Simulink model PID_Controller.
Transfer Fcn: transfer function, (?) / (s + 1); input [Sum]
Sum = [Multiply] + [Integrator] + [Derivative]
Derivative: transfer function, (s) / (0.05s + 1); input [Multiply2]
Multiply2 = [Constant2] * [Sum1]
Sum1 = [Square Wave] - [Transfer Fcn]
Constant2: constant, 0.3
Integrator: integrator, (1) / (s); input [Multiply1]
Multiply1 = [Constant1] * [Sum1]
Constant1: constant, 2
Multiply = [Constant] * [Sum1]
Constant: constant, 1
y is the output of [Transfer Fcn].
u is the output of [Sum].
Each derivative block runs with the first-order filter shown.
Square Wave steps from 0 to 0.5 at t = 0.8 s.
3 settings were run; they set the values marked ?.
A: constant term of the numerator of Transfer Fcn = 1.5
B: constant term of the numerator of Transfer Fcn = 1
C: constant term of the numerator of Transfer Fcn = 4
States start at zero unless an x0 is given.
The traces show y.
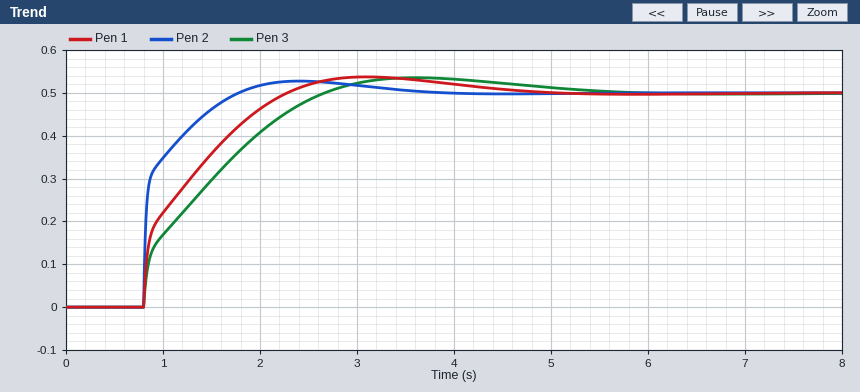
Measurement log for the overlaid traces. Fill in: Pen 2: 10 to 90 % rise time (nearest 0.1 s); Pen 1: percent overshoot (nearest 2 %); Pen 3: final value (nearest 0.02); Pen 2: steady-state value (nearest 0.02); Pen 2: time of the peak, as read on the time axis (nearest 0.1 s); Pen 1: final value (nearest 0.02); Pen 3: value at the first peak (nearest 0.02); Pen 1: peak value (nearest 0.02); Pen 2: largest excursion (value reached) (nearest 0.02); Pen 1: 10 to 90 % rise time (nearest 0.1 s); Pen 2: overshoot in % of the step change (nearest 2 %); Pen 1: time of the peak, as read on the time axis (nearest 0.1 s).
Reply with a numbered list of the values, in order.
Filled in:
1. 0.6 s
2. 8 %
3. 0.50
4. 0.50
5. 2.4 s
6. 0.50
7. 0.54
8. 0.54
9. 0.52
10. 1.1 s
11. 6 %
12. 3.1 s
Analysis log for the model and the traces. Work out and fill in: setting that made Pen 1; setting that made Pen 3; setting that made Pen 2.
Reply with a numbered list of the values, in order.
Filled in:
1. A
2. B
3. C
